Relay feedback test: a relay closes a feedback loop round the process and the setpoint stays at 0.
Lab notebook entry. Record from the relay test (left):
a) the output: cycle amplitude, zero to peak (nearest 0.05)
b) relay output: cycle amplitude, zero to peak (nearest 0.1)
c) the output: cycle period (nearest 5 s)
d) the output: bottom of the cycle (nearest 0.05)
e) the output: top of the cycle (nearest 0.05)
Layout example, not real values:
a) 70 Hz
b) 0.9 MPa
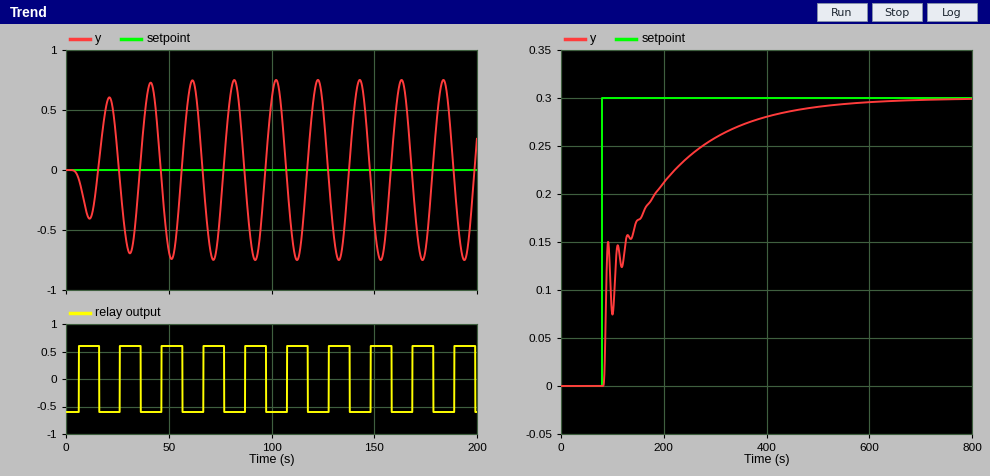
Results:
a) 0.75
b) 0.6
c) 20 s
d) -0.75
e) 0.75
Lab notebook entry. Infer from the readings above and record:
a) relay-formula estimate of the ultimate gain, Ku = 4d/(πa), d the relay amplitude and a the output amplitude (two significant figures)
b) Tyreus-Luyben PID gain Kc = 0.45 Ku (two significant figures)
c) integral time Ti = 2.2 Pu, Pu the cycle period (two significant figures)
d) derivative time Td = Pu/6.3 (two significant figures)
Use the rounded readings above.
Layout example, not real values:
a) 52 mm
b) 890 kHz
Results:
a) 1.0
b) 0.45
c) 44 s
d) 3.2 s
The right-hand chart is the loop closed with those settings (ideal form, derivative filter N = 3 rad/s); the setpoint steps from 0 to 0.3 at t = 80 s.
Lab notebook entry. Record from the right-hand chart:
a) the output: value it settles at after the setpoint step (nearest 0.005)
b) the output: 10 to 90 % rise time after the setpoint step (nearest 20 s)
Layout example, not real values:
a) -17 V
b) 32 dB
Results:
a) 0.300
b) 260 s
